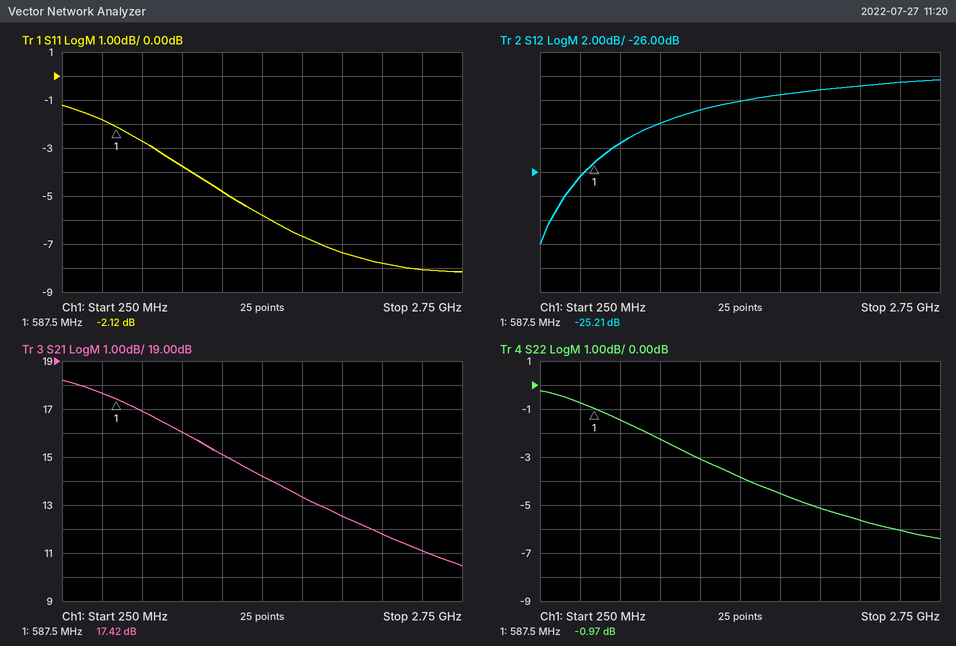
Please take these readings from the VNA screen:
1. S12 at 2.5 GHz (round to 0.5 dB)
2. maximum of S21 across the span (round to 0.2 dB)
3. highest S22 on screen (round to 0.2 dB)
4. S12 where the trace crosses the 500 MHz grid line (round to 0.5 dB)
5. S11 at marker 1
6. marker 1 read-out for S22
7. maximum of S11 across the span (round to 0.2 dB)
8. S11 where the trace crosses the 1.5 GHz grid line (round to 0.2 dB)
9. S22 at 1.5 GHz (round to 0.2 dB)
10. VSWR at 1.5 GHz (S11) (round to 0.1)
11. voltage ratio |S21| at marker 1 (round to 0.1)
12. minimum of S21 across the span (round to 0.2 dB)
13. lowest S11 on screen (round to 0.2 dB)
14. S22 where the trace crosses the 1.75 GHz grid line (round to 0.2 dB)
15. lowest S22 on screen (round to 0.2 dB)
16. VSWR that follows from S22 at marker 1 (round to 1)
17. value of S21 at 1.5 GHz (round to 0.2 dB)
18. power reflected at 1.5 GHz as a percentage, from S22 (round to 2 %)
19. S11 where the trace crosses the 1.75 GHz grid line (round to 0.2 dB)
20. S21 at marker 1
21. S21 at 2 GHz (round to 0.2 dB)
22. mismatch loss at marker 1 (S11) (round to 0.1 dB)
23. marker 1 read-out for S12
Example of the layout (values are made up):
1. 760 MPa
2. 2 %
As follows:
1. -18.5 dB
2. 18.2 dB
3. -0.2 dB
4. -26.5 dB
5. -2.12 dB
6. -0.97 dB
7. -1.2 dB
8. -5.8 dB
9. -3.8 dB
10. 3.1
11. 7.4
12. 10.4 dB
13. -8.2 dB
14. -4.6 dB
15. -6.4 dB
16. 18
17. 14.2 dB
18. 42 %
19. -6.6 dB
20. 17.42 dB
21. 12.6 dB
22. 4.1 dB
23. -25.21 dB
